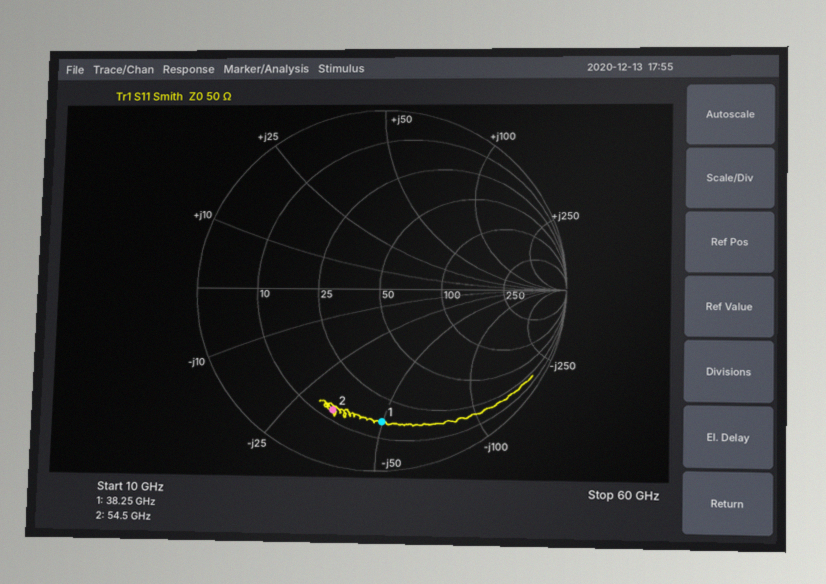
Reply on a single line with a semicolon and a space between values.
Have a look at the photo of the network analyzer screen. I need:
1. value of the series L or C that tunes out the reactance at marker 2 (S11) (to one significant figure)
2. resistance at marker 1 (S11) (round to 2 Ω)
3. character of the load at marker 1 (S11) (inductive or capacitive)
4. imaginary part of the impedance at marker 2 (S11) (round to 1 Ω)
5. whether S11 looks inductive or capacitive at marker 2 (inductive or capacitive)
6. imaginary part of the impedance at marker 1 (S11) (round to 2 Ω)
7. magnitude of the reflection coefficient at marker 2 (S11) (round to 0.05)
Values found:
100 pH; 16 Ω; capacitive; -34 Ω; capacitive; -50 Ω; 0.70
